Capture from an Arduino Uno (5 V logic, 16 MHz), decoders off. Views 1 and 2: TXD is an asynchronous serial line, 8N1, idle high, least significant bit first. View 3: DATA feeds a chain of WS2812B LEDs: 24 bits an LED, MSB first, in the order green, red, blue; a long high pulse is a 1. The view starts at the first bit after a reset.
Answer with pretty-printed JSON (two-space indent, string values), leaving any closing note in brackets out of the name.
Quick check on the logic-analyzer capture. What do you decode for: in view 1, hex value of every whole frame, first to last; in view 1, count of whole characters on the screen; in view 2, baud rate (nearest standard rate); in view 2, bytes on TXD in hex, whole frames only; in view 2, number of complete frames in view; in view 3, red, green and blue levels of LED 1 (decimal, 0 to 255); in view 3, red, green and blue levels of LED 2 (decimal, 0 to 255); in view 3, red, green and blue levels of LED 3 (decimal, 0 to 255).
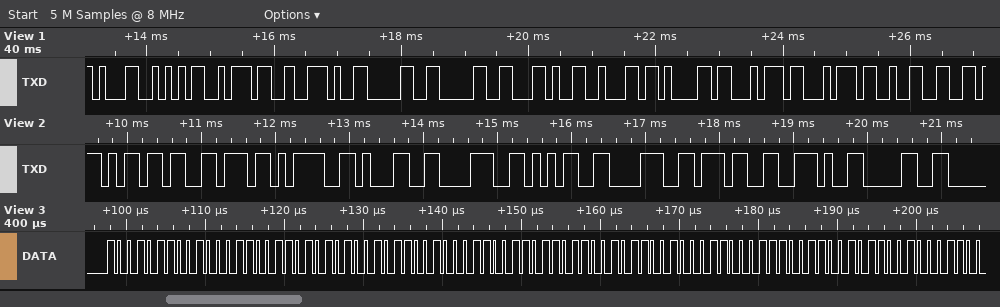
{
  "in view 1, hex value of every whole frame, first to last": "31 35 37 2E 30 30 2C 62 61 74 74 32",
  "in view 1, count of whole characters on the screen": "12",
  "in view 2, baud rate": "9600 baud",
  "in view 2, bytes on TXD in hex, whole frames only": "6D 76 3D 31 38 35 38 37 2E 30",
  "in view 2, number of complete frames in view": "10",
  "in view 3, red, green and blue levels of LED 1": "70, 150, 106",
  "in view 3, red, green and blue levels of LED 2": "70, 150, 109",
  "in view 3, red, green and blue levels of LED 3": "70, 150, 57"
}
